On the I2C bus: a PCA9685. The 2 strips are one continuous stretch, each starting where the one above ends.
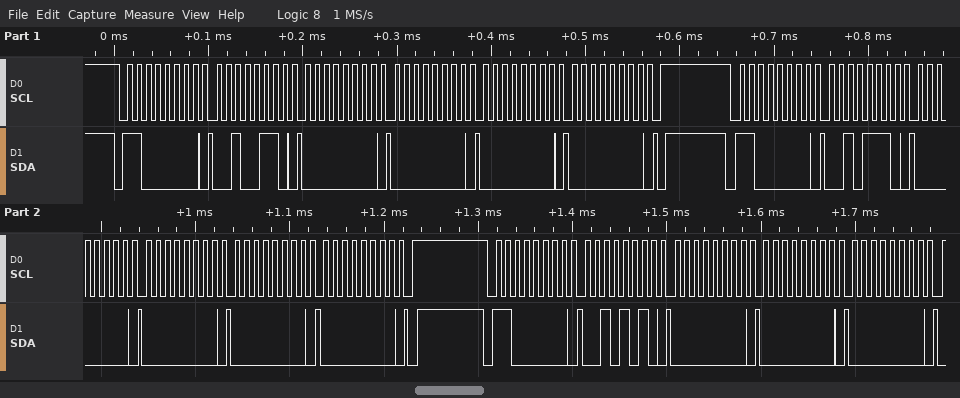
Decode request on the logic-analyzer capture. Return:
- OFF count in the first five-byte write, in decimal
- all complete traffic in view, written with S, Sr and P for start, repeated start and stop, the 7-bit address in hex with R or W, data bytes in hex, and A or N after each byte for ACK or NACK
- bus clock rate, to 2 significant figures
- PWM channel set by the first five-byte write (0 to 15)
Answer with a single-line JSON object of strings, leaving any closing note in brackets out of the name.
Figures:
{"OFF count in the first five-byte write, in decimal": "0", "all complete traffic in view, written with S, Sr and P for start, repeated start and stop, the 7-bit address in hex with R or W, data bytes in hex, and A or N after each byte for ACK or NACK": "S 60W A 26 A 00 A 00 A 00 A 00 A P S 60W A 2E A 00 A 00 A 00 A 00 A P S 60W A 2A A 00 A 00 A 00 A", "bus clock rate, to 2 significant figures": "100 kHz", "PWM channel set by the first five-byte write": "8"}
